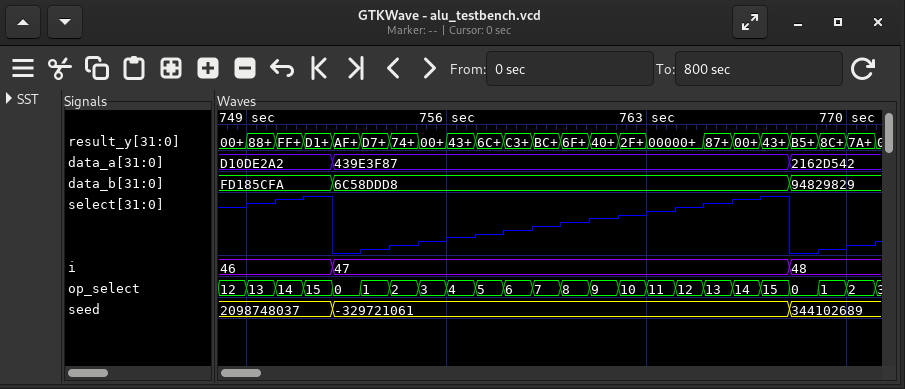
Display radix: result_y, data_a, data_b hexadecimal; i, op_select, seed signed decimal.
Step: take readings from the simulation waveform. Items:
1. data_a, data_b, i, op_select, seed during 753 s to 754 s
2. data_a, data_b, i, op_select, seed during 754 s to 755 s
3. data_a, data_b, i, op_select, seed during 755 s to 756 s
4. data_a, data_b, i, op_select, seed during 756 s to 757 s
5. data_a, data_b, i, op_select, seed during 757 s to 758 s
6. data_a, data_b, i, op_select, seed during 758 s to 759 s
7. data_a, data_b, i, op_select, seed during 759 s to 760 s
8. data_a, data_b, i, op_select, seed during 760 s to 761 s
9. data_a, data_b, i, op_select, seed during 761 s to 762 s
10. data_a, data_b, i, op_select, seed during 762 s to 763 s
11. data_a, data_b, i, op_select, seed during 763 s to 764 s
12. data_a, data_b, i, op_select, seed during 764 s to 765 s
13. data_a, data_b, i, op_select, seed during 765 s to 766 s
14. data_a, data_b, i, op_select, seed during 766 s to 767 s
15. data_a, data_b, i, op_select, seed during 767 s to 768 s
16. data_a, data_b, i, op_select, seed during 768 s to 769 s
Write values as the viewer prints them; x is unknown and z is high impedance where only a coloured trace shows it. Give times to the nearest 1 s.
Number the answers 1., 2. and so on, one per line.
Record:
1. data_a=439E3F87, data_b=6C58DDD8, i=47, op_select=1, seed=-329721061
2. data_a=439E3F87, data_b=6C58DDD8, i=47, op_select=2, seed=-329721061
3. data_a=439E3F87, data_b=6C58DDD8, i=47, op_select=3, seed=-329721061
4. data_a=439E3F87, data_b=6C58DDD8, i=47, op_select=4, seed=-329721061
5. data_a=439E3F87, data_b=6C58DDD8, i=47, op_select=5, seed=-329721061
6. data_a=439E3F87, data_b=6C58DDD8, i=47, op_select=6, seed=-329721061
7. data_a=439E3F87, data_b=6C58DDD8, i=47, op_select=7, seed=-329721061
8. data_a=439E3F87, data_b=6C58DDD8, i=47, op_select=8, seed=-329721061
9. data_a=439E3F87, data_b=6C58DDD8, i=47, op_select=9, seed=-329721061
10. data_a=439E3F87, data_b=6C58DDD8, i=47, op_select=10, seed=-329721061
11. data_a=439E3F87, data_b=6C58DDD8, i=47, op_select=11, seed=-329721061
12. data_a=439E3F87, data_b=6C58DDD8, i=47, op_select=12, seed=-329721061
13. data_a=439E3F87, data_b=6C58DDD8, i=47, op_select=13, seed=-329721061
14. data_a=439E3F87, data_b=6C58DDD8, i=47, op_select=14, seed=-329721061
15. data_a=439E3F87, data_b=6C58DDD8, i=47, op_select=15, seed=-329721061
16. data_a=2162D542, data_b=94829829, i=48, op_select=0, seed=344102689
